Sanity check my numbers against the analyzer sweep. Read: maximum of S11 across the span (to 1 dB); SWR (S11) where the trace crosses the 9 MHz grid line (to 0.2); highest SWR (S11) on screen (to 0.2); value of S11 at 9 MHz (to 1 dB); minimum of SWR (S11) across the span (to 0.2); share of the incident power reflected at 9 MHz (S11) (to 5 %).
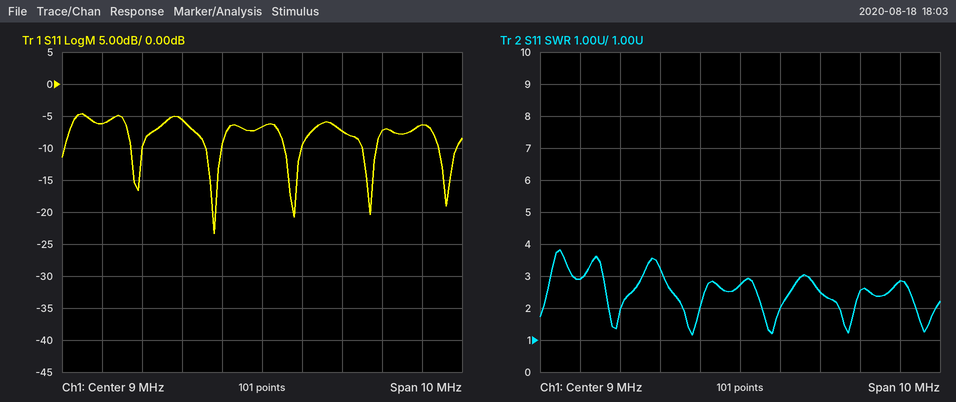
-5 dB
2.8
3.8
-7 dB
1.2
20 %
